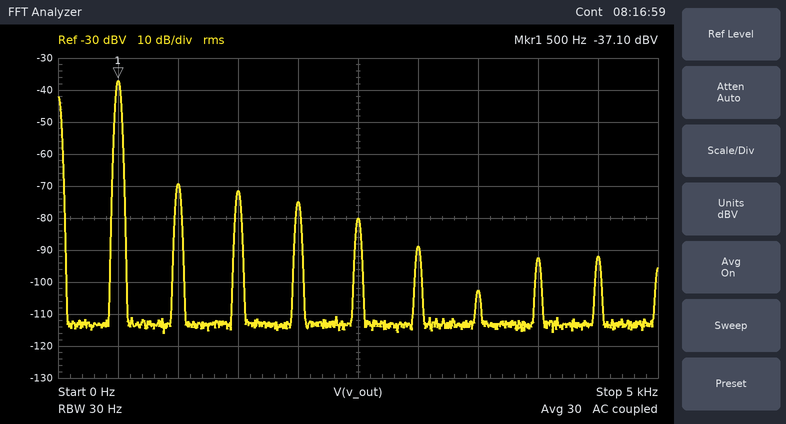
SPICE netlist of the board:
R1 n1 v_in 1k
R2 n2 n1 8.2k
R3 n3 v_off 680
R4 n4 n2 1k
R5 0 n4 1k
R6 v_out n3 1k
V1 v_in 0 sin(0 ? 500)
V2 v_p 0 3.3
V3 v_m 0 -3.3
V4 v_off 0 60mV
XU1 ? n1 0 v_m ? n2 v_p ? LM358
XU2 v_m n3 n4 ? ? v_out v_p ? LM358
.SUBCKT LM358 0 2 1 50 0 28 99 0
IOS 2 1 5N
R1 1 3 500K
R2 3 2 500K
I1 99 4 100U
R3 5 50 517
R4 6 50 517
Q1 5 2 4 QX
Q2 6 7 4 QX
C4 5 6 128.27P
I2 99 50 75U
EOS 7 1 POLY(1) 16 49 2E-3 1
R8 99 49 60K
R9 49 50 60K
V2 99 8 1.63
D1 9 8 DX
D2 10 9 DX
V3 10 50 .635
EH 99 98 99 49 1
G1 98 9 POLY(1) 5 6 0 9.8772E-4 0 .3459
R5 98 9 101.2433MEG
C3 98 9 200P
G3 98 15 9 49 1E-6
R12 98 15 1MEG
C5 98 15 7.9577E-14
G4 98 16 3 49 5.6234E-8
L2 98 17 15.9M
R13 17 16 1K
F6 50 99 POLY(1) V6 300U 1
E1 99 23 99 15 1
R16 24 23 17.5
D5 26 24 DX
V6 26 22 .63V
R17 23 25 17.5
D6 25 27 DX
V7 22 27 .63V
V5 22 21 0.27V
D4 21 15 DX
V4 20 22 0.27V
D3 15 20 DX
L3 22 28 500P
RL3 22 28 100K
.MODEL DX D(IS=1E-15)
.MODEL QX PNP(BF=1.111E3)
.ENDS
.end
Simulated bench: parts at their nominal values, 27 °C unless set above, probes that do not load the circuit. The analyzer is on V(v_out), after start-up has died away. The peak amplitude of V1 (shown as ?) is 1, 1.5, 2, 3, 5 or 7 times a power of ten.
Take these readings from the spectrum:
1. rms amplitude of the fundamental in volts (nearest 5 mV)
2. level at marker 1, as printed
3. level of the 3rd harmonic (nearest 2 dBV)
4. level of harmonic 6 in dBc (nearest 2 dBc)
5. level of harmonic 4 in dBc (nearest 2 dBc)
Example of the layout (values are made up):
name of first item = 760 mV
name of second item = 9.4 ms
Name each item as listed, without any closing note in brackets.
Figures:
rms amplitude of the fundamental in volts = 15 mV
level at marker 1, as printed = -37.10 dBV
level of the 3rd harmonic = -72 dBV
level of harmonic 6 in dBc = -52 dBc
level of harmonic 4 in dBc = -38 dBc
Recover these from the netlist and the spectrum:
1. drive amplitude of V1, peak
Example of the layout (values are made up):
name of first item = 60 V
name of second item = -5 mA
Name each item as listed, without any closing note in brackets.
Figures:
drive amplitude of V1, peak = 2 mV
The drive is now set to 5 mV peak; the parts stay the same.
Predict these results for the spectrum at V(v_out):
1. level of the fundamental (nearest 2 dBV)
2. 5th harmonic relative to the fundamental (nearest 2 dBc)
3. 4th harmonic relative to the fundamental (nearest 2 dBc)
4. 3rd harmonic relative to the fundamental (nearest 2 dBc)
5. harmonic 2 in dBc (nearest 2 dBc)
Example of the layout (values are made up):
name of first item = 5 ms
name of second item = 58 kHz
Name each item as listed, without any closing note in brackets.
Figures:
level of the fundamental = -30 dBV
5th harmonic relative to the fundamental = -36 dBc
4th harmonic relative to the fundamental = -42 dBc
3rd harmonic relative to the fundamental = -28 dBc
harmonic 2 in dBc = -18 dBc
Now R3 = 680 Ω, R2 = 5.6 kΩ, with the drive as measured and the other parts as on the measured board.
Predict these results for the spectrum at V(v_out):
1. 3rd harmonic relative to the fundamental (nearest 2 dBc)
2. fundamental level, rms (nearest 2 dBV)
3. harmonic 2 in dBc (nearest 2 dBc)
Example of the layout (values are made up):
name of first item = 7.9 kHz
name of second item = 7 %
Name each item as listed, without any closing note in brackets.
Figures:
3rd harmonic relative to the fundamental = -32 dBc
fundamental level, rms = -40 dBV
harmonic 2 in dBc = -28 dBc
